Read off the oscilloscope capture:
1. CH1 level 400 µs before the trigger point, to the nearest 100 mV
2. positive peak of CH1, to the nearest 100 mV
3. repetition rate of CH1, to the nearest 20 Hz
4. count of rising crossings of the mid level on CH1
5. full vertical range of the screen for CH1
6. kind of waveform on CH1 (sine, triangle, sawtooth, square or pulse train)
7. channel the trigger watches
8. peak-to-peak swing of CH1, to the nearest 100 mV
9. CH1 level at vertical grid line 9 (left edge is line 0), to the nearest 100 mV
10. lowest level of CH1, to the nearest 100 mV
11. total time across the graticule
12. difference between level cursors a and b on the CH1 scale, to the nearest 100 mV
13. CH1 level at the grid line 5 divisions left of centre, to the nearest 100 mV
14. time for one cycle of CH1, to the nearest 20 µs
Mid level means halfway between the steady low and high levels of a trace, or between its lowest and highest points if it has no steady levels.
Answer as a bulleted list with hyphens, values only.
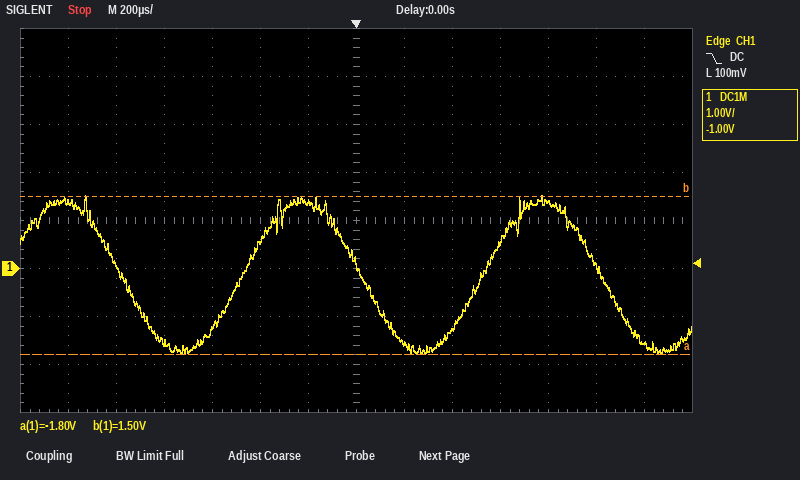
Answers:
- 600 mV
- 1.5 V
- 1.00 kHz
- 2
- 8 V
- sine
- CH1
- 3.3 V
- -1.3 V
- -1.8 V
- 2.8 ms
- 3.3 V
- 100 mV
- 1.00 ms
